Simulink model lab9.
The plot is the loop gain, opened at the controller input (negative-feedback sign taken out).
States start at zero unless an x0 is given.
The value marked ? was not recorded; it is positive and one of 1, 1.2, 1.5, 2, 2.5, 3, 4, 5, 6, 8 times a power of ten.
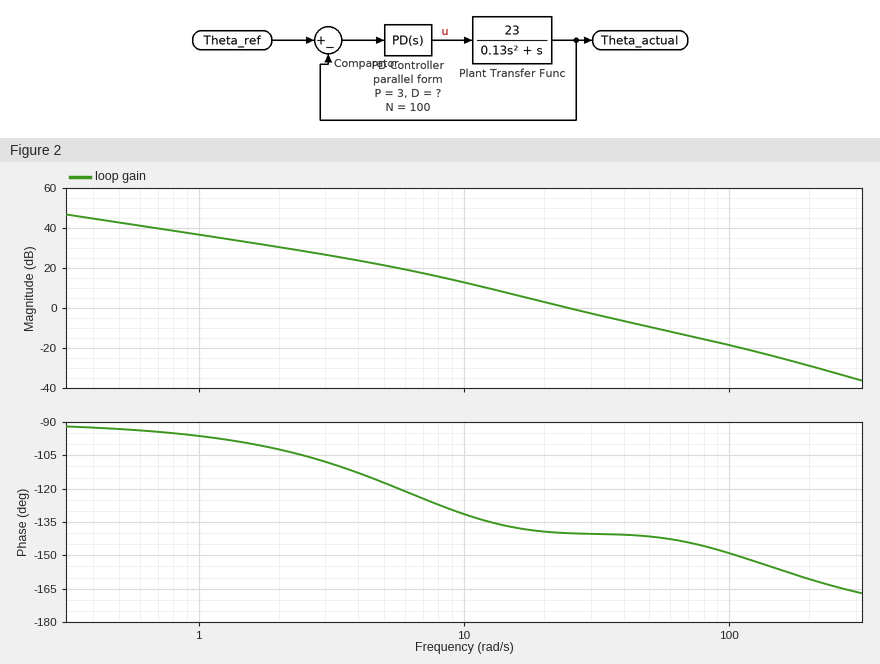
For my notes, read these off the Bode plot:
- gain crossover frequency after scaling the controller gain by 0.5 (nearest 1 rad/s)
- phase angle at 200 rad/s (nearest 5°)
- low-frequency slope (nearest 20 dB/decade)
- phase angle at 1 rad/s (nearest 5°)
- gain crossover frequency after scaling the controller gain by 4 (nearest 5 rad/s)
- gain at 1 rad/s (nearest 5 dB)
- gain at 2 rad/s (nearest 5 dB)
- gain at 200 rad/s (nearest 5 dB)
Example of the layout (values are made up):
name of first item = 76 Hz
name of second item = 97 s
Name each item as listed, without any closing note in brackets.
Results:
gain crossover frequency after scaling the controller gain by 0.5 = 16 rad/s
phase angle at 200 rad/s = -160°
low-frequency slope = -20 dB/decade
phase angle at 1 rad/s = -95°
gain crossover frequency after scaling the controller gain by 4 = 60 rad/s
gain at 1 rad/s = 35 dB
gain at 2 rad/s = 30 dB
gain at 200 rad/s = -30 dB
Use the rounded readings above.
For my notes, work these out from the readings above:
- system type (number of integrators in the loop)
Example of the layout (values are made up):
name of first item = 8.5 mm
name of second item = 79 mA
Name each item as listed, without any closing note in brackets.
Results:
system type = 1
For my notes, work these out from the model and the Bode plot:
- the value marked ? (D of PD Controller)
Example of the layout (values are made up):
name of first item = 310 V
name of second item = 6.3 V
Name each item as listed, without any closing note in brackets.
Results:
the value marked ? = 0.06
